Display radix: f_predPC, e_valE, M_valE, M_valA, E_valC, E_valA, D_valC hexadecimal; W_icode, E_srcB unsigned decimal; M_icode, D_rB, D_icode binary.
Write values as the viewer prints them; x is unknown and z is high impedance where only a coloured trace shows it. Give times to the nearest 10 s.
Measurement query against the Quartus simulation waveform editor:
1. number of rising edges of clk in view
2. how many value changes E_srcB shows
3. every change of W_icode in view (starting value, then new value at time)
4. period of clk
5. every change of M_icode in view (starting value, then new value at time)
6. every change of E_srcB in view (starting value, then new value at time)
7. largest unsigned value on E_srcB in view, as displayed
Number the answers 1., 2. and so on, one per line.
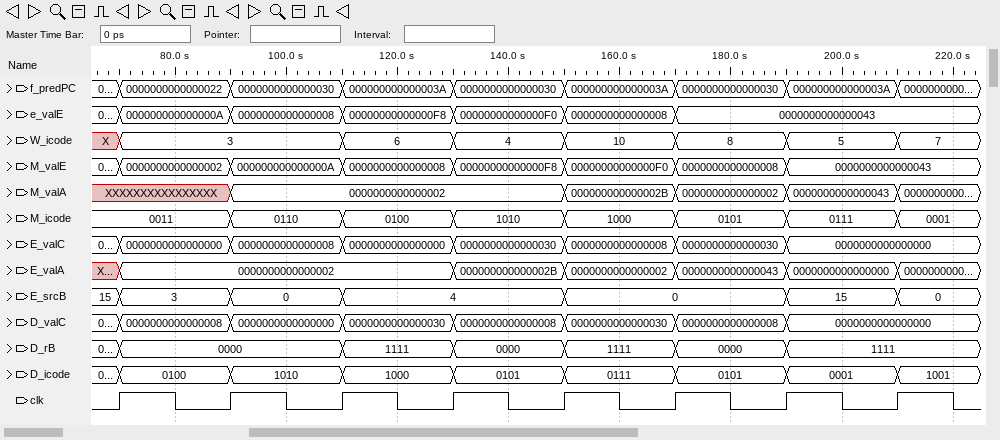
1. 8
2. 6
3. X, 3 at 70 s, 6 at 110 s, 4 at 130 s, 10 at 150 s, 8 at 170 s, 5 at 190 s, 7 at 210 s
4. 20 s
5. 0011, 0110 at 90 s, 0100 at 110 s, 1010 at 130 s, 1000 at 150 s, 0101 at 170 s, 0111 at 190 s, 0001 at 210 s
6. 15, 3 at 70 s, 0 at 90 s, 4 at 110 s, 0 at 150 s, 15 at 190 s, 0 at 210 s
7. 15
